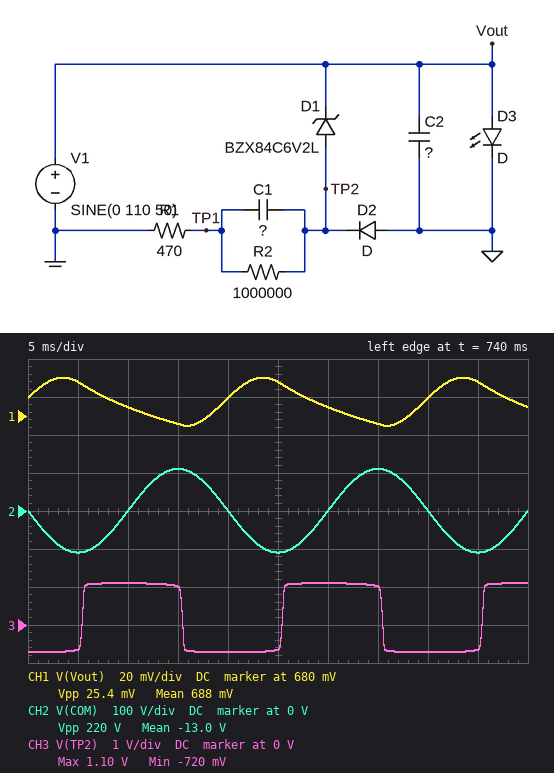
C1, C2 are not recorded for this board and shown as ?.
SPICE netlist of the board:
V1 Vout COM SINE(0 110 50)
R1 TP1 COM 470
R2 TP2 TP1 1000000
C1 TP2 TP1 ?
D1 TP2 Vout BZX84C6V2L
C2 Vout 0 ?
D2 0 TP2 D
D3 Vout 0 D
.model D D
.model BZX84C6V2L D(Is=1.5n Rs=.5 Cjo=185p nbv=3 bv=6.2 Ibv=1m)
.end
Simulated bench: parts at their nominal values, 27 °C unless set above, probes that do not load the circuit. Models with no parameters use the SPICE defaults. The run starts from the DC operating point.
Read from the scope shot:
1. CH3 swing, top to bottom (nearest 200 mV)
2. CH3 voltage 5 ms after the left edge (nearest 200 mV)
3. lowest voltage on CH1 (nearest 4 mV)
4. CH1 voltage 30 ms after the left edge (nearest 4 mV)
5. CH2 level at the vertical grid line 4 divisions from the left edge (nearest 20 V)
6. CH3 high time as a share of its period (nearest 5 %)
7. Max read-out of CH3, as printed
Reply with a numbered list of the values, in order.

1. 1.8 V
2. -600 mV
3. 676 mV
4. 684 mV
5. 0 V
6. 50 %
7. 1.10 V
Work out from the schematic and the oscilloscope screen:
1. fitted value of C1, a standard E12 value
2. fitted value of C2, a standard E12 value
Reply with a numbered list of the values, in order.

1. 330 nF
2. 1.5 mF
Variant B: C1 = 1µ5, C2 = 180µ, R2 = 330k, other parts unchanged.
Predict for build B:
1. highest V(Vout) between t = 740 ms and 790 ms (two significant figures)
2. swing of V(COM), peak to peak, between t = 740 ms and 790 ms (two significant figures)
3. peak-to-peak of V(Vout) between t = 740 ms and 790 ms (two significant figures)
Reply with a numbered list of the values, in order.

1. 760 mV
2. 220 V
3. 120 mV
